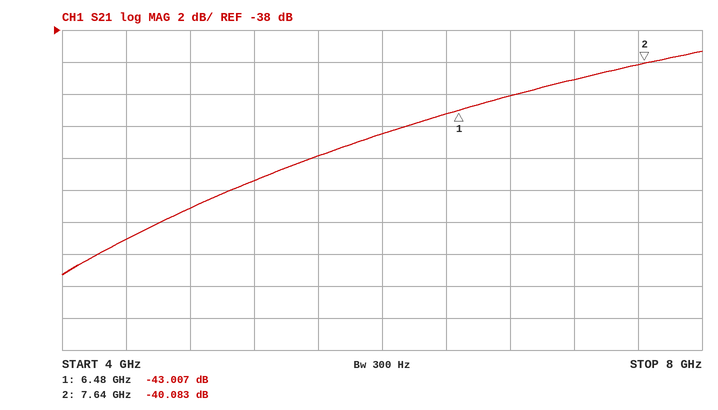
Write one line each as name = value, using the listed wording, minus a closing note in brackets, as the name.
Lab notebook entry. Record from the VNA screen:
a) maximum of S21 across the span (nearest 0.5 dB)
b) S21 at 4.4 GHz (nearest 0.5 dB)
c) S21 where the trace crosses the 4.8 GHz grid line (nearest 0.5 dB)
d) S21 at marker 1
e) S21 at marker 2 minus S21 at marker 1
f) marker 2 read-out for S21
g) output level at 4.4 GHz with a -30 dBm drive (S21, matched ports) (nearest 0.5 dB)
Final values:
maximum of S21 across the span = -39.5 dB
S21 at 4.4 GHz = -51.0 dB
S21 where the trace crosses the 4.8 GHz grid line = -49.0 dB
S21 at marker 1 = -43.007 dB
S21 at marker 2 minus S21 at marker 1 = 2.924 dB
marker 2 read-out for S21 = -40.083 dB
output level at 4.4 GHz with a -30 dBm drive (S21, matched ports) = -81.0 dBm
